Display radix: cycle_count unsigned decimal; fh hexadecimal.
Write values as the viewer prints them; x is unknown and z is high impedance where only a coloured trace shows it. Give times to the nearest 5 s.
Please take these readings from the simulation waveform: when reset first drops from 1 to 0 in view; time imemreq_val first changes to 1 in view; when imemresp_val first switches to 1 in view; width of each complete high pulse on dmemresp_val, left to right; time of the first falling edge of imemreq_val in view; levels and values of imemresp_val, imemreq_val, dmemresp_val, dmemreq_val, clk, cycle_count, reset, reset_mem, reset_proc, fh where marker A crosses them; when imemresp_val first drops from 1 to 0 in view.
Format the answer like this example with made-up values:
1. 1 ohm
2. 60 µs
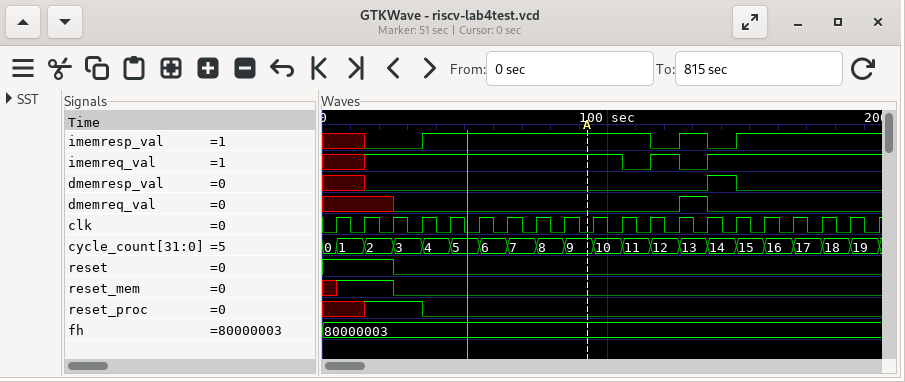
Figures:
1. 25 s
2. 15 s
3. 35 s
4. 10 s
5. 105 s
6. imemresp_val=1, imemreq_val=1, dmemresp_val=0, dmemreq_val=0, clk=0, cycle_count=9, reset=0, reset_mem=0, reset_proc=0, fh=80000003
7. 115 s
